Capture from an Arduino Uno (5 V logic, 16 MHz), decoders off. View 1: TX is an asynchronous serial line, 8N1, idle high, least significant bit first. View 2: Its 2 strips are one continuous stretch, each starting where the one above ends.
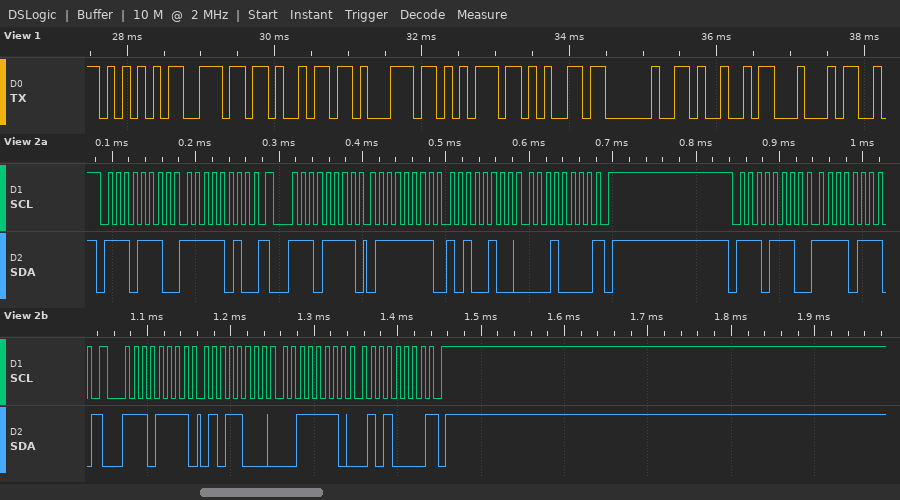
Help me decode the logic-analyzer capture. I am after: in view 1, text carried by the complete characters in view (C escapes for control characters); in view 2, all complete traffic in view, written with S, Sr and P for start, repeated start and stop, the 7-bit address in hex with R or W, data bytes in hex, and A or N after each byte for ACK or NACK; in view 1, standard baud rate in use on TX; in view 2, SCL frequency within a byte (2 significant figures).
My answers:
"Unique ID"
S 77W A FA A Sr 77R A 7F A A4 A 10 N P S 77W A F7 A Sr 77R A 58 A 3E A 50 N P
9600 baud
100 kHz
